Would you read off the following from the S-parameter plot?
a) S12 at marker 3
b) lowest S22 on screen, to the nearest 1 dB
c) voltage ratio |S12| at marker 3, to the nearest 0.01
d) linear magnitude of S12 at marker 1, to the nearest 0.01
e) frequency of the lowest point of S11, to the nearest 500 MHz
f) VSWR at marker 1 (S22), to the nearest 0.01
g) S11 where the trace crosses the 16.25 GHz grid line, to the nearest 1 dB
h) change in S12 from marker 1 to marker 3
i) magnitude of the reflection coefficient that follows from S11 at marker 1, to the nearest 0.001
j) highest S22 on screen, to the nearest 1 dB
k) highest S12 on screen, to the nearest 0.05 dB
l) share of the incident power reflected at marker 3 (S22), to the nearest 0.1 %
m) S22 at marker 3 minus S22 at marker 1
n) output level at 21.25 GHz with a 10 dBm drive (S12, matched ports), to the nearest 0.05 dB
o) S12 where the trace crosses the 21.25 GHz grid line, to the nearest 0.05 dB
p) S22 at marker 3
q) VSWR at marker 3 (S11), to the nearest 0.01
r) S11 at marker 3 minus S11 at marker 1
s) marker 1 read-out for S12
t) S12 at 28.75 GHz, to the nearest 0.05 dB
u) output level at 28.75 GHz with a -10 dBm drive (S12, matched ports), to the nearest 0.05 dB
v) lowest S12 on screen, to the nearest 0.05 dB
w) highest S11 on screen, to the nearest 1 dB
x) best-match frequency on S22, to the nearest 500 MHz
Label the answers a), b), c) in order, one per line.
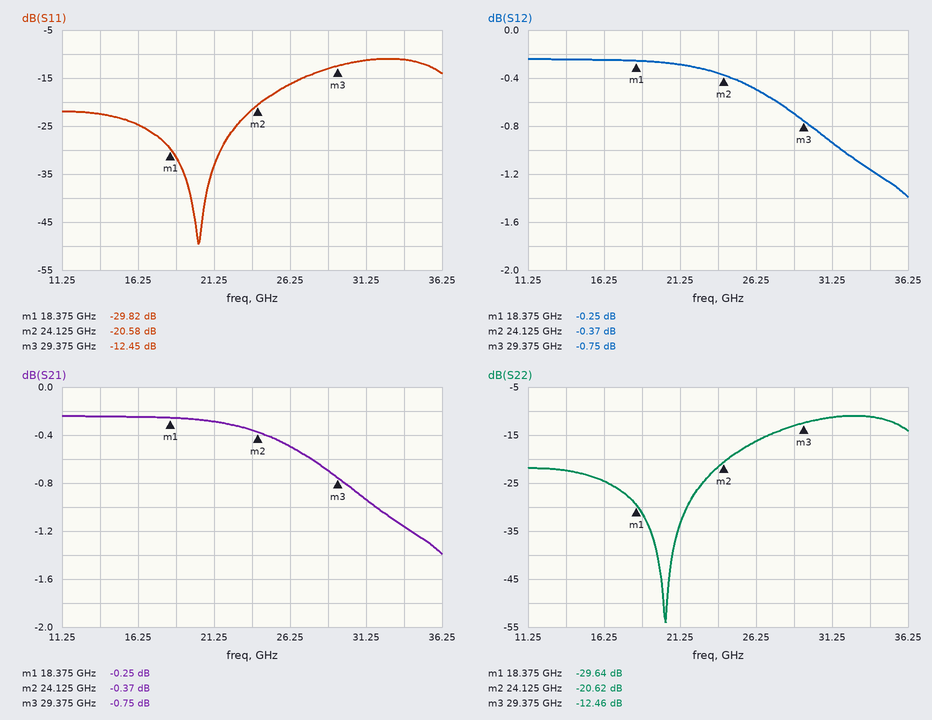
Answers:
a) -0.75 dB
b) -54 dB
c) 0.92
d) 0.97
e) 20.0 GHz
f) 1.07
g) -25 dB
h) -0.50 dB
i) 0.032
j) -11 dB
k) -0.25 dB
l) 5.7 %
m) 17.18 dB
n) 9.70 dBm
o) -0.30 dB
p) -12.46 dB
q) 1.63
r) 17.37 dB
s) -0.25 dB
t) -0.70 dB
u) -10.70 dBm
v) -1.40 dB
w) -11 dB
x) 20.5 GHz
